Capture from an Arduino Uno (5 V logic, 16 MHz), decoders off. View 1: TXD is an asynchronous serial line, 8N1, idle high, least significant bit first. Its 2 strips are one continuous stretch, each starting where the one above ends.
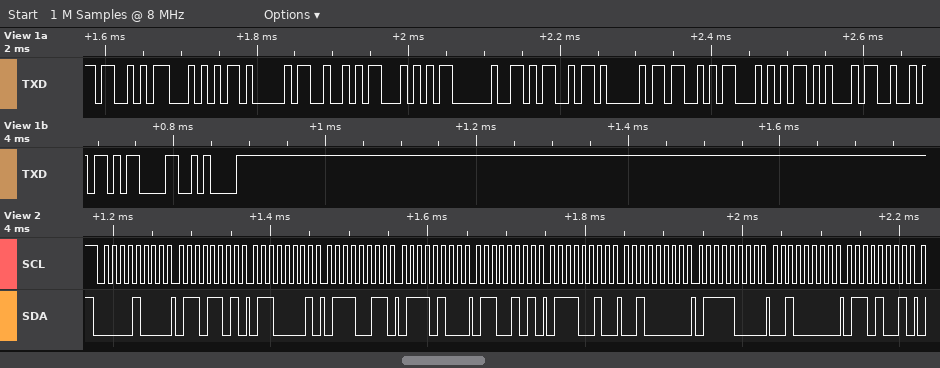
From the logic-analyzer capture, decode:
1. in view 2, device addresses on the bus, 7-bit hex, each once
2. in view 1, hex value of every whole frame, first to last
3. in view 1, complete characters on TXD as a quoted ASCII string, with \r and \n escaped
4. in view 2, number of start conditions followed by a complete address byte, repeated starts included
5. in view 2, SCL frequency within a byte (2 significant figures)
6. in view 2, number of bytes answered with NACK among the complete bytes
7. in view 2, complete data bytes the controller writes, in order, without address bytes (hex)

0x04
53 54 41 52 54 20 4D 41 53 54 45 52 0D 0A
"START MASTER\r\n"
1
100 kHz
0
6D 61 73 74 65 72 20 78 20 69
